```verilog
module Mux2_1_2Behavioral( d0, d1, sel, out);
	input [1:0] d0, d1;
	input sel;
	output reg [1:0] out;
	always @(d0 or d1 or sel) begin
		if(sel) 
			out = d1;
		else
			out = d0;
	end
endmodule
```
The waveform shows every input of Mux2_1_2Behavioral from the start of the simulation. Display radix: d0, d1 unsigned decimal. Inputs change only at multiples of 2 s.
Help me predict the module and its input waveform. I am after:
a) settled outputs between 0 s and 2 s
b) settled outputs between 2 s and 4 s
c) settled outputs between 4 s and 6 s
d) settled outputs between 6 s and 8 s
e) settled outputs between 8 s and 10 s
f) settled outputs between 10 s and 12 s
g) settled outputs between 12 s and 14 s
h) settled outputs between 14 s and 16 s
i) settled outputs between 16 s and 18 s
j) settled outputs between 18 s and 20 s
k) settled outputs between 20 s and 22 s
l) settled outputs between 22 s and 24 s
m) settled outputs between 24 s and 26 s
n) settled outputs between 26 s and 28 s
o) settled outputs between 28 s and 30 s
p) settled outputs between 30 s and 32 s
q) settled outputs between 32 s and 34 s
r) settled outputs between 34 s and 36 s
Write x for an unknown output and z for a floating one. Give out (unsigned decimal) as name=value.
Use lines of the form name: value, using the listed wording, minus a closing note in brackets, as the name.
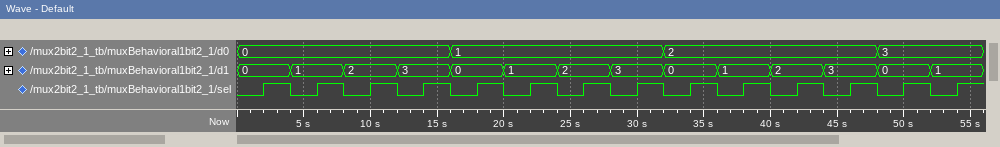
settled outputs between 0 s and 2 s: out=0
settled outputs between 2 s and 4 s: out=0
settled outputs between 4 s and 6 s: out=0
settled outputs between 6 s and 8 s: out=1
settled outputs between 8 s and 10 s: out=0
settled outputs between 10 s and 12 s: out=2
settled outputs between 12 s and 14 s: out=0
settled outputs between 14 s and 16 s: out=3
settled outputs between 16 s and 18 s: out=1
settled outputs between 18 s and 20 s: out=0
settled outputs between 20 s and 22 s: out=1
settled outputs between 22 s and 24 s: out=1
settled outputs between 24 s and 26 s: out=1
settled outputs between 26 s and 28 s: out=2
settled outputs between 28 s and 30 s: out=1
settled outputs between 30 s and 32 s: out=3
settled outputs between 32 s and 34 s: out=2
settled outputs between 34 s and 36 s: out=0
